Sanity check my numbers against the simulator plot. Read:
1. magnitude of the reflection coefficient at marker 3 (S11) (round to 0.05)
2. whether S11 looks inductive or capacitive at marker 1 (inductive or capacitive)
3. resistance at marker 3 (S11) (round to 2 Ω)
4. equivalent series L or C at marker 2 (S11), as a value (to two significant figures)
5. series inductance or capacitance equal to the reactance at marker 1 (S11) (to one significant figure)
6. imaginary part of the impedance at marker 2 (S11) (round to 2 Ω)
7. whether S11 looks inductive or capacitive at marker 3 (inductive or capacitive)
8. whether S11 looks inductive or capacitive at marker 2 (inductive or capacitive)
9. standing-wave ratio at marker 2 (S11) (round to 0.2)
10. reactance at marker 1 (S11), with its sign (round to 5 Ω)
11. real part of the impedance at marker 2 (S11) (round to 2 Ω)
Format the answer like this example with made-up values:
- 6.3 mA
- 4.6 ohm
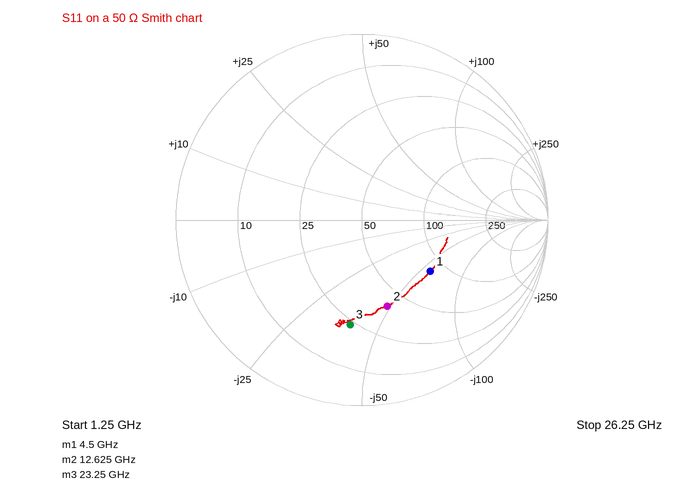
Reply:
- 0.55
- capacitive
- 24 Ω
- 260 fF
- 600 fF
- -48 Ω
- capacitive
- capacitive
- 2.8
- -60 Ω
- 40 Ω
